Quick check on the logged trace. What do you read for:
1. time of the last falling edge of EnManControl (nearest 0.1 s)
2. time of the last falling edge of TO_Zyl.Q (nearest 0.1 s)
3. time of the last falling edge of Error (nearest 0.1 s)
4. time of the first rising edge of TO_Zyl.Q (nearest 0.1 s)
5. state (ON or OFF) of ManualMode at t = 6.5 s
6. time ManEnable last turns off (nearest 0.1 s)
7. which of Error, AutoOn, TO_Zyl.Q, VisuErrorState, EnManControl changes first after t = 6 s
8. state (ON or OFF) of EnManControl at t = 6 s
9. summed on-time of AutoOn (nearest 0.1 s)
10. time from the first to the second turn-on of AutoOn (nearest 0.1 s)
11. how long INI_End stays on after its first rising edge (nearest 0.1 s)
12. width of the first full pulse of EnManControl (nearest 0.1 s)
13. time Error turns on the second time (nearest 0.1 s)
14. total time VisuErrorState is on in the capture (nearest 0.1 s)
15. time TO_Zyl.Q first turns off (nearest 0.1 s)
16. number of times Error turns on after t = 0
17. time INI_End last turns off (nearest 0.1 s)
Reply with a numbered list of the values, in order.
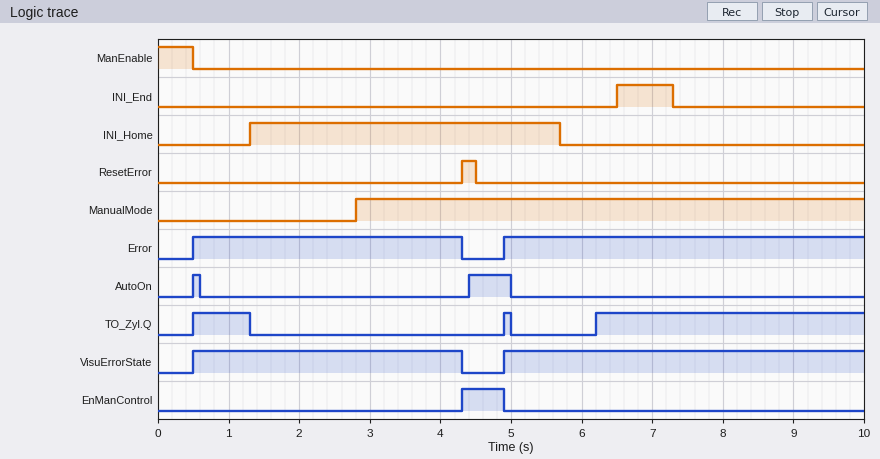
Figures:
1. 4.9 s
2. 5.0 s
3. 4.3 s
4. 0.5 s
5. ON
6. 0.5 s
7. TO_Zyl.Q
8. OFF
9. 0.7 s
10. 3.9 s
11. 0.8 s
12. 0.6 s
13. 4.9 s
14. 8.9 s
15. 1.3 s
16. 2
17. 7.3 s
